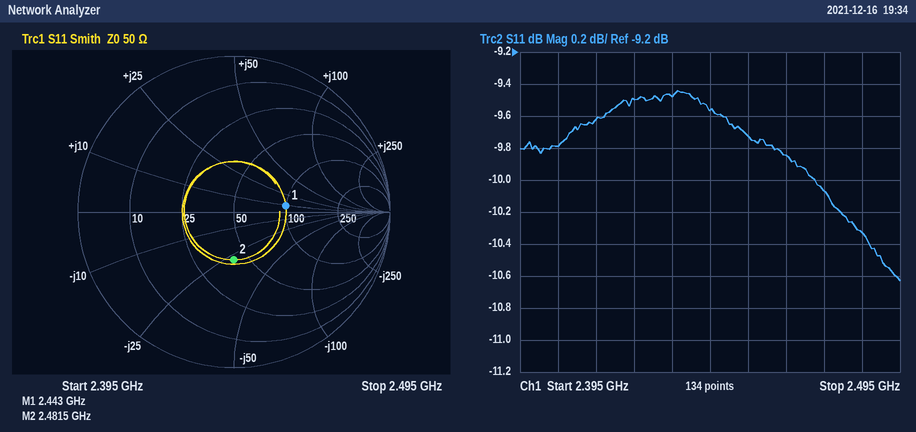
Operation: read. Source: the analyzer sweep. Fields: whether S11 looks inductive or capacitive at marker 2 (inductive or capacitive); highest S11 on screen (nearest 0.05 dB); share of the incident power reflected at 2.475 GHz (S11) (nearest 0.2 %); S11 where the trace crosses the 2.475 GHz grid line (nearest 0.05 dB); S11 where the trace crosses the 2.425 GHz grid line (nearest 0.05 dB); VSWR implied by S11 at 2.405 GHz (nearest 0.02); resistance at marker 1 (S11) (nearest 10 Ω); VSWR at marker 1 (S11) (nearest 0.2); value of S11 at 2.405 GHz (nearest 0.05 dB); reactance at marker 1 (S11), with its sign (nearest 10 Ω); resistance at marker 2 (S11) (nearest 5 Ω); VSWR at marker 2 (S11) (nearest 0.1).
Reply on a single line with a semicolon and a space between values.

capacitive; -9.45 dB; 9.8 %; -10.05 dB; -9.50 dB; 1.96; 100 Ω; 2.0; -9.80 dB; +10 Ω; 40 Ω; 1.9
